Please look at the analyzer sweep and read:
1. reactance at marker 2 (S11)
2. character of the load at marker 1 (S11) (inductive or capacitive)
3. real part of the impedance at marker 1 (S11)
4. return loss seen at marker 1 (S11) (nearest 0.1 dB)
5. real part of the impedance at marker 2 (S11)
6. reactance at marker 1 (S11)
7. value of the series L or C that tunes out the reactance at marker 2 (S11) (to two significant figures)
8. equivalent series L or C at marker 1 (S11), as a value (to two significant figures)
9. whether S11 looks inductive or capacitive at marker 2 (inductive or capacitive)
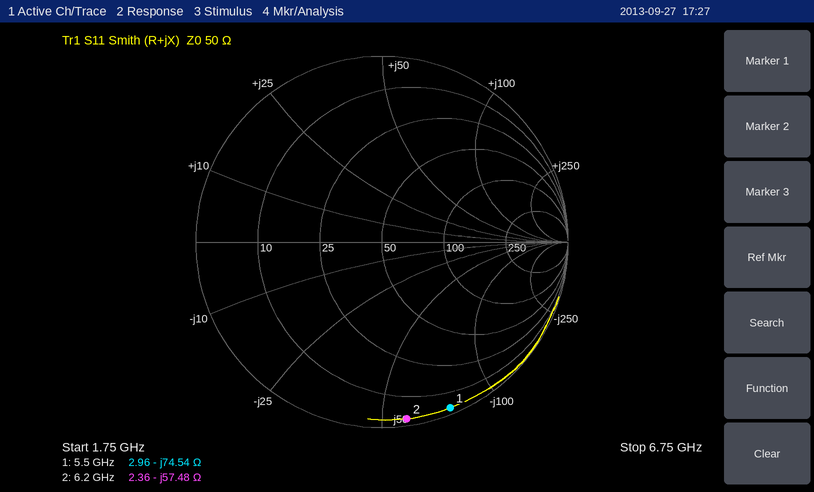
-57.48 Ω
capacitive
2.96 Ω
0.3 dB
2.36 Ω
-74.54 Ω
1.5 nH
390 fF
capacitive
